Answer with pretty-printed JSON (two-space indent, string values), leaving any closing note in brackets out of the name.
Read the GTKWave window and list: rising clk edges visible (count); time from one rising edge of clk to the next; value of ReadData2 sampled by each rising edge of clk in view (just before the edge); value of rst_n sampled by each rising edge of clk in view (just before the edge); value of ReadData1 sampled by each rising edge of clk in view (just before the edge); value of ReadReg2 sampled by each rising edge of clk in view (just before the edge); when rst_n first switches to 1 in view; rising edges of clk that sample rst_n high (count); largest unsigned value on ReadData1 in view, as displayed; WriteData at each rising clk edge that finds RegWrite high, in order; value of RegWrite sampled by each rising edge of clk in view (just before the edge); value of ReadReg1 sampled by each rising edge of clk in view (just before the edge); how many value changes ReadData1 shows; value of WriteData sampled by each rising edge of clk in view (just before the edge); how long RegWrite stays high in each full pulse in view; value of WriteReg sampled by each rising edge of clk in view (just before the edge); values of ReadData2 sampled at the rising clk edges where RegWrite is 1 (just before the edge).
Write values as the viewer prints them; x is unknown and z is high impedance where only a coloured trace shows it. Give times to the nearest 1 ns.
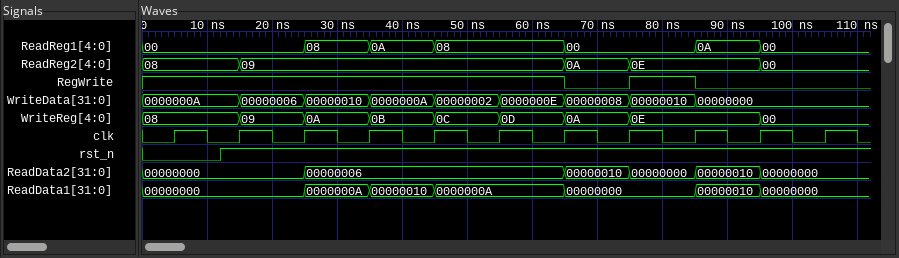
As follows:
{
  "rising clk edges visible": "11",
  "time from one rising edge of clk to the next": "10 ns",
  "value of ReadData2 sampled by each rising edge of clk in view": "00000000, 00000000, 00000000, 00000006, 00000006, 00000006, 00000006, 00000010, 00000000, 00000010, 00000000",
  "value of rst_n sampled by each rising edge of clk in view": "0 1 1 1 1 1 1 1 1 1 1",
  "value of ReadData1 sampled by each rising edge of clk in view": "00000000, 00000000, 00000000, 0000000A, 00000010, 0000000A, 0000000A, 00000000, 00000000, 00000010, 00000000",
  "value of ReadReg2 sampled by each rising edge of clk in view": "08, 08, 09, 09, 09, 09, 09, 0A, 0E, 0E, 00",
  "when rst_n first switches to 1 in view": "12 ns",
  "rising edges of clk that sample rst_n high": "10",
  "largest unsigned value on ReadData1 in view, as displayed": "00000010",
  "WriteData at each rising clk edge that finds RegWrite high, in order": "0000000A, 0000000A, 00000006, 00000010, 0000000A, 00000002, 0000000E, 00000010",
  "value of RegWrite sampled by each rising edge of clk in view": "1 1 1 1 1 1 1 0 1 0 0",
  "value of ReadReg1 sampled by each rising edge of clk in view": "00, 00, 00, 08, 0A, 08, 08, 00, 00, 0A, 00",
  "how many value changes ReadData1 shows": "6",
  "value of WriteData sampled by each rising edge of clk in view": "0000000A, 0000000A, 00000006, 00000010, 0000000A, 00000002, 0000000E, 00000008, 00000010, 00000000, 00000000",
  "how long RegWrite stays high in each full pulse in view": "10 ns",
  "value of WriteReg sampled by each rising edge of clk in view": "08, 08, 09, 0A, 0B, 0C, 0D, 0A, 0E, 0E, 00",
  "values of ReadData2 sampled at the rising clk edges where RegWrite is 1": "00000000, 00000000, 00000000, 00000006, 00000006, 00000006, 00000006, 00000000"
}
